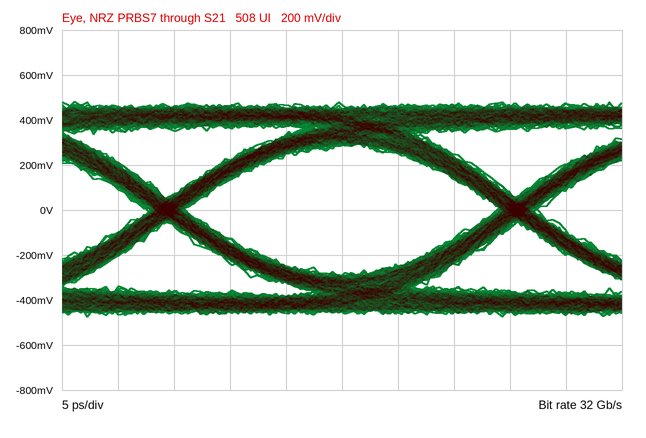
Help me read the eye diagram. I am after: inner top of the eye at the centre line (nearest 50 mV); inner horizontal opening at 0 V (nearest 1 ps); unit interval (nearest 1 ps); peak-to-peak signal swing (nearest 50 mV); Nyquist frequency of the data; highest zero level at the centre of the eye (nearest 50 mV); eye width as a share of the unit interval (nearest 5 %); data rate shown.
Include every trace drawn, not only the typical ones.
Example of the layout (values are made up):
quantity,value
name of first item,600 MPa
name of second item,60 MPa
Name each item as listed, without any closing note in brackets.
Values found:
quantity,value
inner top of the eye at the centre line,300 mV
inner horizontal opening at 0 V,28 ps
unit interval,31 ps
peak-to-peak signal swing,950 mV
Nyquist frequency of the data,16 GHz
highest zero level at the centre of the eye,-300 mV
eye width as a share of the unit interval,90 %
data rate shown,32 Gb/s
